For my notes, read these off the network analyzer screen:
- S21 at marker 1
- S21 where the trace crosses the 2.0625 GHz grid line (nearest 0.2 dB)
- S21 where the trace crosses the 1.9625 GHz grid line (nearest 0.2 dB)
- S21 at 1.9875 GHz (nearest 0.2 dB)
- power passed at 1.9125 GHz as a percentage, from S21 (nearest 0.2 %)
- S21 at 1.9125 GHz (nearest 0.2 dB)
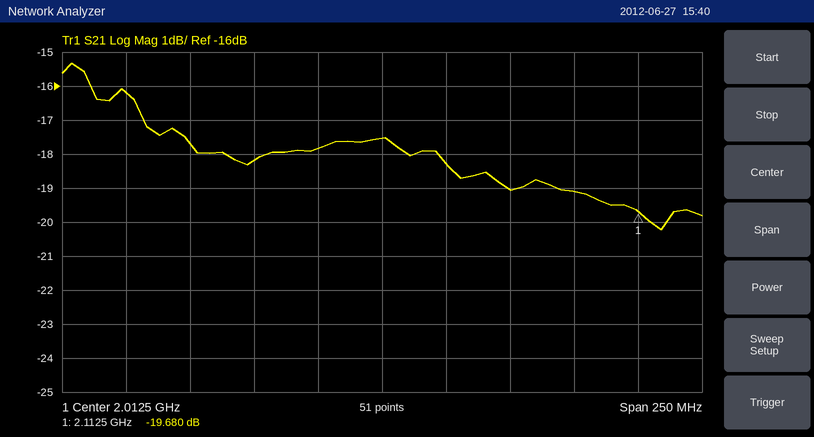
-19.680 dB
-19.0 dB
-18.2 dB
-17.8 dB
2.4 %
-16.2 dB
